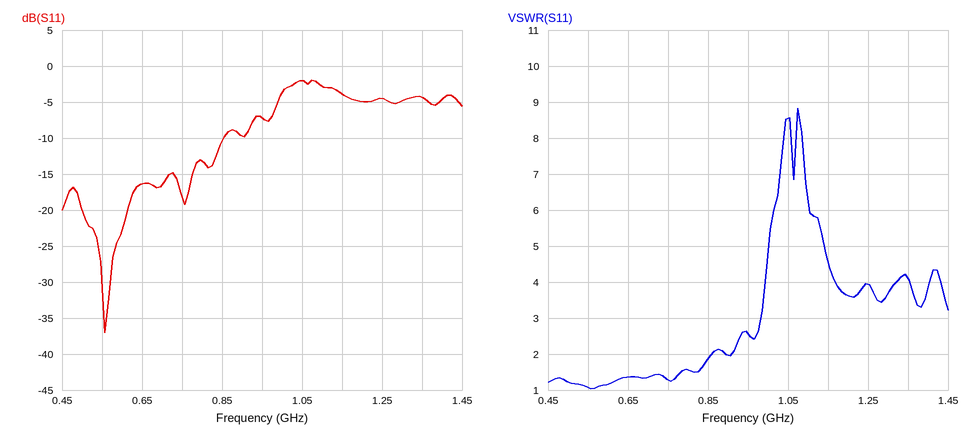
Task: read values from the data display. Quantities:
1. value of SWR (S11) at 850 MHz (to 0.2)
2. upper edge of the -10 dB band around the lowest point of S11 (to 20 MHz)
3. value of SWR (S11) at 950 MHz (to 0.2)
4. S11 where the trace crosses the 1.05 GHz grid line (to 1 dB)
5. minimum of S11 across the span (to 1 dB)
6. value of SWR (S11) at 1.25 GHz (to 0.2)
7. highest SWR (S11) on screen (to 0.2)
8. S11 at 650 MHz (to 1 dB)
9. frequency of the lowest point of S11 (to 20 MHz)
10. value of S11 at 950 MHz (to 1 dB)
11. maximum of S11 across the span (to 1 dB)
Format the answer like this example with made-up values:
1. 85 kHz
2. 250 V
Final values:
1. 1.8
2. 860 MHz
3. 2.6
4. -2 dB
5. -37 dB
6. 4.0
7. 8.8
8. -16 dB
9. 560 MHz
10. -7 dB
11. -2 dB
